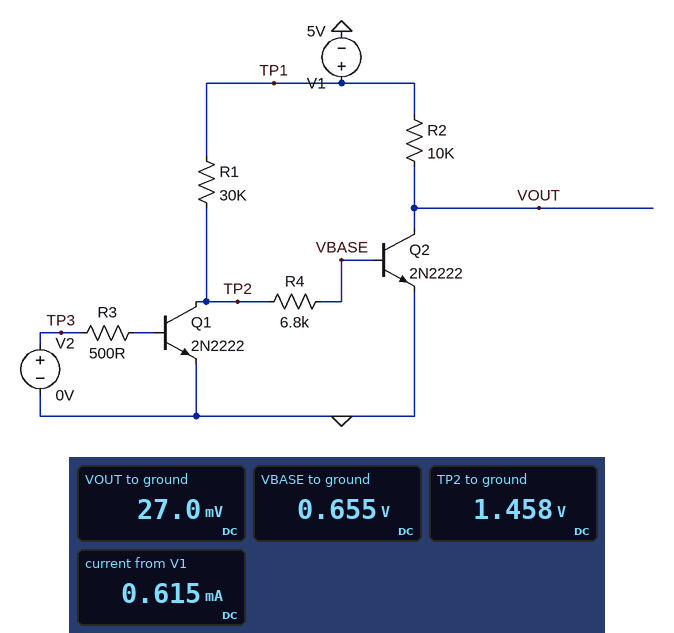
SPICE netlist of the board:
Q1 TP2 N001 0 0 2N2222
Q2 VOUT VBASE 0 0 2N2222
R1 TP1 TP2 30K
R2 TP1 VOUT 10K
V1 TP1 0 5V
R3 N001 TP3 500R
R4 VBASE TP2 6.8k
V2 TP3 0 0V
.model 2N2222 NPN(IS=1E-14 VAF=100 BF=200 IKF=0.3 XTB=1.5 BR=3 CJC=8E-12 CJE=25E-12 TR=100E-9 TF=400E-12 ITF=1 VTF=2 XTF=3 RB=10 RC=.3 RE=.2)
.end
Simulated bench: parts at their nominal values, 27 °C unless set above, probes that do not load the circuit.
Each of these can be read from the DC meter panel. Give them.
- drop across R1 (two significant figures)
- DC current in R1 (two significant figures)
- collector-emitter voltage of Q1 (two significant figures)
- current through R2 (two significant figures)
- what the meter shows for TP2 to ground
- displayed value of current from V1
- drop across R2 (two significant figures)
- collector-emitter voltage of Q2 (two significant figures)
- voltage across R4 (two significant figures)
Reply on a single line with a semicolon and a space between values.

3.5 V; 120 µA; 1.5 V; 500 µA; 1.458 V; 0.615 mA; 5.0 V; 27 mV; 800 mV
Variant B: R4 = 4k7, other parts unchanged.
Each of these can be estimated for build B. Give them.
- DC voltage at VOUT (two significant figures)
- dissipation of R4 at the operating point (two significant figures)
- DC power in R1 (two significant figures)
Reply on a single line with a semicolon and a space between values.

26 mV; 74 µW; 470 µW
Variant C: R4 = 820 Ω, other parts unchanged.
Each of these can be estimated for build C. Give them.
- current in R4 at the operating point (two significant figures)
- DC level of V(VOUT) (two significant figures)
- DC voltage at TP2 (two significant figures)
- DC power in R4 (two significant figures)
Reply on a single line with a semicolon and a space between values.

140 µA; 25 mV; 770 mV; 16 µW
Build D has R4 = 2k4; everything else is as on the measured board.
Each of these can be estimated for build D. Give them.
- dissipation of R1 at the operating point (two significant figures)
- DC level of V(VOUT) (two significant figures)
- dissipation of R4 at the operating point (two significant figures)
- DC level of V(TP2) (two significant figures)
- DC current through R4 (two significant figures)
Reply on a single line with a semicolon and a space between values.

540 µW; 25 mV; 43 µW; 980 mV; 130 µA
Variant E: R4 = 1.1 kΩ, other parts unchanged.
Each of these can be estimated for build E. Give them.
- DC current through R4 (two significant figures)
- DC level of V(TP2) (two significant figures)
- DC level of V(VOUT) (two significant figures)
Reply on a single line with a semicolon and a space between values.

140 µA; 810 mV; 25 mV
